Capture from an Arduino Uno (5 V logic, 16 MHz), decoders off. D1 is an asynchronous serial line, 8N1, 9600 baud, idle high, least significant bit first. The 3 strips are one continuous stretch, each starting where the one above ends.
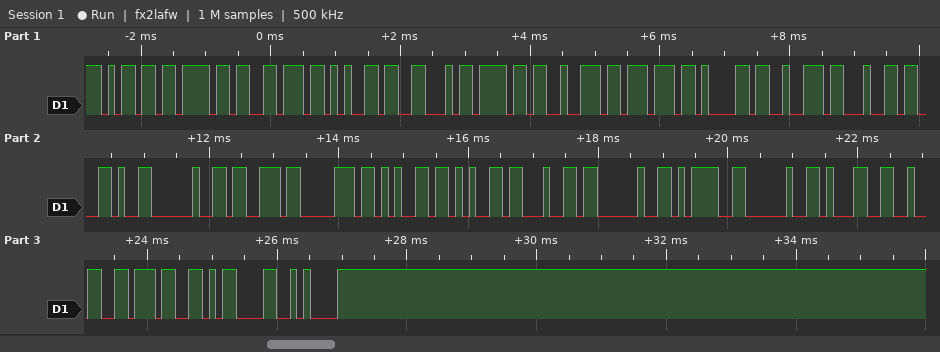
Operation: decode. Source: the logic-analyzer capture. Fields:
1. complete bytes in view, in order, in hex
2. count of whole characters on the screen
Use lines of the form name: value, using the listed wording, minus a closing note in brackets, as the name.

complete bytes in view, in order, in hex: 6D 6F 76 65 46 6F 72 77 61 72 64 2C 20 73 70 65 65 64 20 3D 20 31 32 37 0D 0A
count of whole characters on the screen: 26
